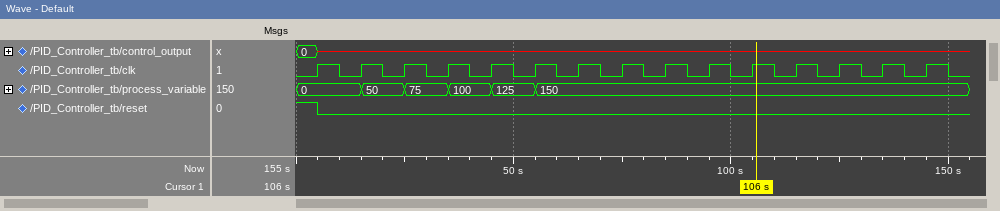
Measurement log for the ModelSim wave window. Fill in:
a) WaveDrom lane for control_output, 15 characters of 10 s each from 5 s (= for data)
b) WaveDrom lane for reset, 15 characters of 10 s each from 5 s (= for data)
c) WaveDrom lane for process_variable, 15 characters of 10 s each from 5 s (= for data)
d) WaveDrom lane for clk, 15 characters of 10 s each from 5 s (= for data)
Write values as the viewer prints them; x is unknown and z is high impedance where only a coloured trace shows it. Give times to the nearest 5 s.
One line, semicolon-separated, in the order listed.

{name: 'control_output', wave: 'x..............'}; {name: 'reset', wave: '0..............'}; {name: 'process_variable', wave: '======.........', data: '0 50 75 100 125 150'}; {name: 'clk', wave: 'p..............'}
